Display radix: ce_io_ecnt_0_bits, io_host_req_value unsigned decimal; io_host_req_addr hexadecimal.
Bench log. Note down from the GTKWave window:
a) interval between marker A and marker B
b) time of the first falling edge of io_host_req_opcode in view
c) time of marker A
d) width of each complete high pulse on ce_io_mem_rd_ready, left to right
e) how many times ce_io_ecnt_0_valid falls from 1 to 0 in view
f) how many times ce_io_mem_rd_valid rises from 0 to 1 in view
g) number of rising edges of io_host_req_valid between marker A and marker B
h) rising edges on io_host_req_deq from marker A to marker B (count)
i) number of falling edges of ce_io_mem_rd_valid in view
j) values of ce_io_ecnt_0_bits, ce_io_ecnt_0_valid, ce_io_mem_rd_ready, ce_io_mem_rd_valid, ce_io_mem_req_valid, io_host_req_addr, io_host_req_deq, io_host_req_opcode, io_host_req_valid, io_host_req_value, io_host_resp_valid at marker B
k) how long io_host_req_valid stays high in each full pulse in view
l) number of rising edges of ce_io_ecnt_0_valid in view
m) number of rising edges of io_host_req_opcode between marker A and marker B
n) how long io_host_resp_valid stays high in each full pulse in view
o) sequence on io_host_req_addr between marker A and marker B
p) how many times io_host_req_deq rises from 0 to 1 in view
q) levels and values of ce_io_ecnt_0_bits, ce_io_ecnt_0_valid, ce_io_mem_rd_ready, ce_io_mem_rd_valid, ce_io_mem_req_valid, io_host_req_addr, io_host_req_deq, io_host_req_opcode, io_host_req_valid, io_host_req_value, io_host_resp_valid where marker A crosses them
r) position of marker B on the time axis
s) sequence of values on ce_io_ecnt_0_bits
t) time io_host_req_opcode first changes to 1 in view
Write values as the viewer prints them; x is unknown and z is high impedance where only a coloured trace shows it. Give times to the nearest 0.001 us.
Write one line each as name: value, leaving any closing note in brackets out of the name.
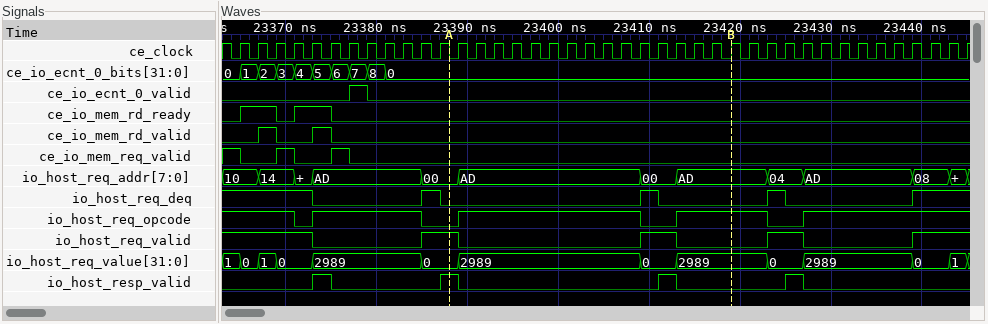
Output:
interval between marker A and marker B: 0.031 us
time of the first falling edge of io_host_req_opcode in view: 23.371 us
time of marker A: 23.388 us
width of each complete high pulse on ce_io_mem_rd_ready, left to right: 0.004 us, 0.004 us
how many times ce_io_ecnt_0_valid falls from 1 to 0 in view: 1
how many times ce_io_mem_rd_valid rises from 0 to 1 in view: 2
number of rising edges of io_host_req_valid between marker A and marker B: 1
rising edges on io_host_req_deq from marker A to marker B: 1
number of falling edges of ce_io_mem_rd_valid in view: 2
values of ce_io_ecnt_0_bits, ce_io_ecnt_0_valid, ce_io_mem_rd_ready, ce_io_mem_rd_valid, ce_io_mem_req_valid, io_host_req_addr, io_host_req_deq, io_host_req_opcode, io_host_req_valid, io_host_req_value, io_host_resp_valid at marker B: ce_io_ecnt_0_bits=0, ce_io_ecnt_0_valid=0, ce_io_mem_rd_ready=0, ce_io_mem_rd_valid=0, ce_io_mem_req_valid=0, io_host_req_addr=AD, io_host_req_deq=0, io_host_req_opcode=1, io_host_req_valid=0, io_host_req_value=2989, io_host_resp_valid=0
how long io_host_req_valid stays high in each full pulse in view: 0.004 us, 0.004 us, 0.004 us
number of rising edges of ce_io_ecnt_0_valid in view: 1
number of rising edges of io_host_req_opcode between marker A and marker B: 2
how long io_host_resp_valid stays high in each full pulse in view: 0.002 us, 0.002 us, 0.002 us, 0.002 us
sequence on io_host_req_addr between marker A and marker B: 00, AD, 00, AD
how many times io_host_req_deq rises from 0 to 1 in view: 4
levels and values of ce_io_ecnt_0_bits, ce_io_ecnt_0_valid, ce_io_mem_rd_ready, ce_io_mem_rd_valid, ce_io_mem_req_valid, io_host_req_addr, io_host_req_deq, io_host_req_opcode, io_host_req_valid, io_host_req_value, io_host_resp_valid where marker A crosses them: ce_io_ecnt_0_bits=0, ce_io_ecnt_0_valid=0, ce_io_mem_rd_ready=0, ce_io_mem_rd_valid=0, ce_io_mem_req_valid=0, io_host_req_addr=00, io_host_req_deq=0, io_host_req_opcode=0, io_host_req_valid=1, io_host_req_value=0, io_host_resp_valid=1
position of marker B on the time axis: 23.419 us
sequence of values on ce_io_ecnt_0_bits: 0, 1, 2, 3, 4, 5, 6, 7, 8, 0
time io_host_req_opcode first changes to 1 in view: 23.373 us
